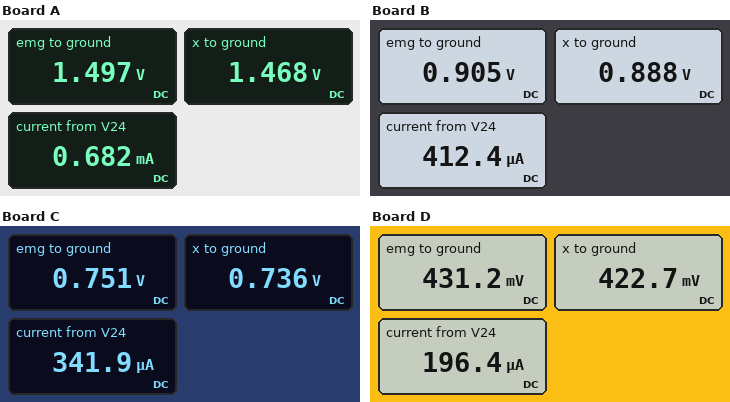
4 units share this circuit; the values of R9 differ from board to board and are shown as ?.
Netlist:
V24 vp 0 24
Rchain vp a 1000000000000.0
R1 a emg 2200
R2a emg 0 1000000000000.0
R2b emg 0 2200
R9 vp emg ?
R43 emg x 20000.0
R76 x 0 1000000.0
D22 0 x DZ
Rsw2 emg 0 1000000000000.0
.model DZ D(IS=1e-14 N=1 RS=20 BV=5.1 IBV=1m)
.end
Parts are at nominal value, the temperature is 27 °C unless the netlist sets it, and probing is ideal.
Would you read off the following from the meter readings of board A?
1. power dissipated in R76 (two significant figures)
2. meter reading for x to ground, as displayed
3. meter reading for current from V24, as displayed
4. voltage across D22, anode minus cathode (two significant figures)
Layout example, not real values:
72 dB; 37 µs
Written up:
2.2 µW; 1.468 V; 0.682 mA; -1.5 V
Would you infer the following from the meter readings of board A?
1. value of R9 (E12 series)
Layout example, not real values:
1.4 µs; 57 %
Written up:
33 kΩ
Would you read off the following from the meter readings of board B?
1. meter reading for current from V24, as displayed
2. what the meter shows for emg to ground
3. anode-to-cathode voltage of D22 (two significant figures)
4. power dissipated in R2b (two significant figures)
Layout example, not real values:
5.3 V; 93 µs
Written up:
412.4 µA; 0.905 V; -890 mV; 370 µW
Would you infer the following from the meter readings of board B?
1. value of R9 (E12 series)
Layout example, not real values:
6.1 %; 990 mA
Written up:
56 kΩ
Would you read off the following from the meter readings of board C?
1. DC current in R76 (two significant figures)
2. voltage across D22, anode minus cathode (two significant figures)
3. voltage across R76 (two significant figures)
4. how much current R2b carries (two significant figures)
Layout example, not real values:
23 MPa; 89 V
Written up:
740 nA; -740 mV; 740 mV; 340 µA
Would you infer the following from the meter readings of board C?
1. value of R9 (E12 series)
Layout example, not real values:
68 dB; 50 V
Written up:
68 kΩ
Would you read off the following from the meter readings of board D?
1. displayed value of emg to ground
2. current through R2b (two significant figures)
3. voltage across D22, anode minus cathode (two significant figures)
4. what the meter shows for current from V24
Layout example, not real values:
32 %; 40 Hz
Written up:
431.2 mV; 200 µA; -420 mV; 196.4 µA
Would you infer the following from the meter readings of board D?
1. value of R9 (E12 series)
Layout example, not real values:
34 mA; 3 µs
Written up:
120 kΩ
